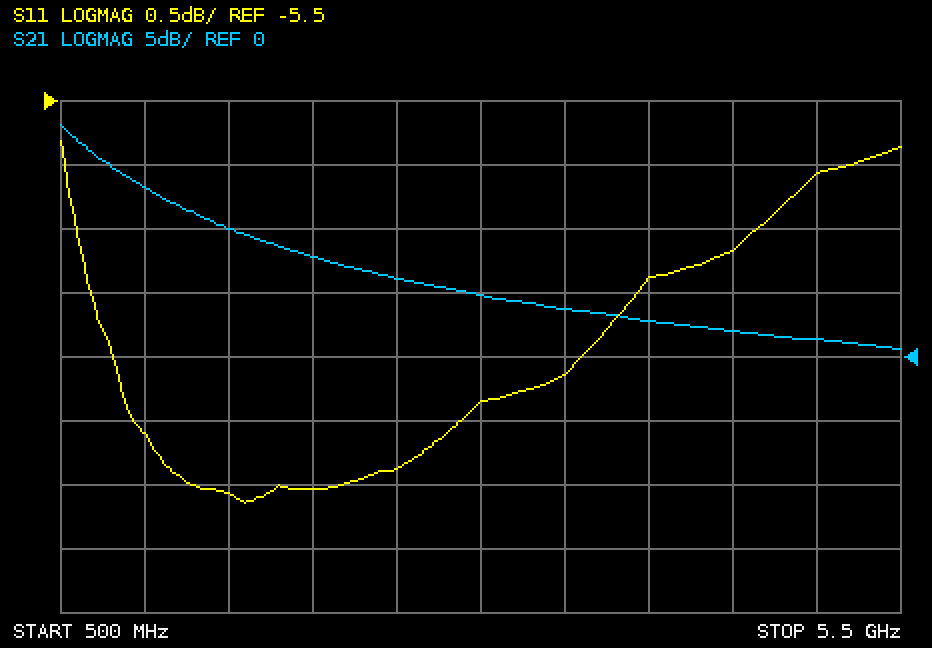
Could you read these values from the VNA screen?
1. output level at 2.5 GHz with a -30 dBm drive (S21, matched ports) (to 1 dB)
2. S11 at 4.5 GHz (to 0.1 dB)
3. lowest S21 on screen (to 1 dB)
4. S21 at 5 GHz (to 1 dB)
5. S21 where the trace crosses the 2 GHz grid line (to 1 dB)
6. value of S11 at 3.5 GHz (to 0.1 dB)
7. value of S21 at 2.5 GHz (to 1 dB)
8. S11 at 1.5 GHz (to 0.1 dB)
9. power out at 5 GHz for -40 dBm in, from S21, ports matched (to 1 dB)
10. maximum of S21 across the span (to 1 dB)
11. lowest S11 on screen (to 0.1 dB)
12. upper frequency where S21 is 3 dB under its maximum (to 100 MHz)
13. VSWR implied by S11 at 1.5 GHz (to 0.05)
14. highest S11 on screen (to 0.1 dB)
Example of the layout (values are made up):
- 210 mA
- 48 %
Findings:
- -24 dBm
- -6.7 dB
- 1 dB
- 1 dB
- 8 dB
- -7.6 dB
- 6 dB
- -8.6 dB
- -39 dBm
- 18 dB
- -8.6 dB
- 800 MHz
- 2.20
- -5.8 dB
